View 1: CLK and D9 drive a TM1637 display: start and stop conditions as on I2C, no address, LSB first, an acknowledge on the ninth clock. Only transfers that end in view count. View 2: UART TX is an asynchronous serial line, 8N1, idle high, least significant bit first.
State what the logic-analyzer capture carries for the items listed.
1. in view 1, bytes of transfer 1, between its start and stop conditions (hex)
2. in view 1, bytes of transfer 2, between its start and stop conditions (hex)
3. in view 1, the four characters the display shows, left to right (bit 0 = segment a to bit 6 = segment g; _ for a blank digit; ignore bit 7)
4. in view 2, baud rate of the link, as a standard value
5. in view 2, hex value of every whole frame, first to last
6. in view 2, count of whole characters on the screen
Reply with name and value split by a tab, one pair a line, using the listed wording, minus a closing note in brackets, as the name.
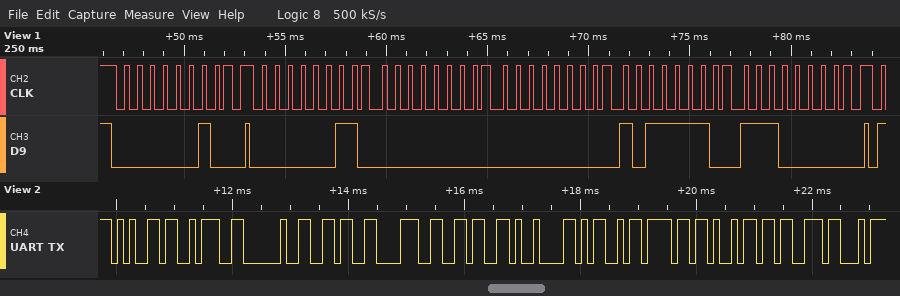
in view 1, bytes of transfer 1, between its start and stop conditions	40
in view 1, bytes of transfer 2, between its start and stop conditions	C0 00 00 7D 07
in view 1, the four characters the display shows, left to right	__67
in view 2, baud rate of the link, as a standard value	9600 baud
in view 2, hex value of every whole frame, first to last	65 3A 20 36 38 36 09 4D 6F 69 73
in view 2, count of whole characters on the screen	11
